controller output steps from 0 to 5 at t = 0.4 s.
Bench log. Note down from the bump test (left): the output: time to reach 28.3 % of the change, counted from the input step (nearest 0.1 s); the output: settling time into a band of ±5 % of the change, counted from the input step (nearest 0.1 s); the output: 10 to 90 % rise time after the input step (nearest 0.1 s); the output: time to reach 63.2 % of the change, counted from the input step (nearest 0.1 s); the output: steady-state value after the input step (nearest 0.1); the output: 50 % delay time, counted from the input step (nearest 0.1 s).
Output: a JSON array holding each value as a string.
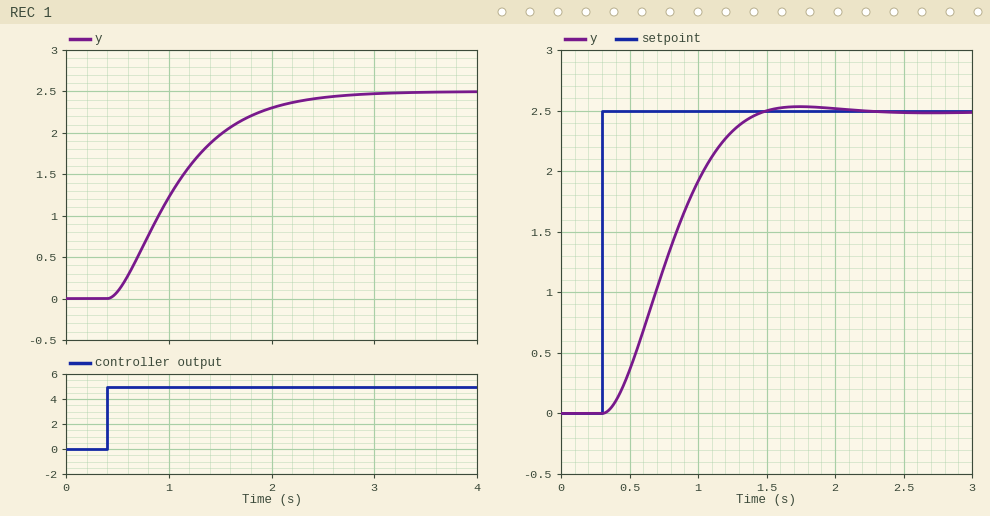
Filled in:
["0.4 s", "1.8 s", "1.3 s", "0.8 s", "2.5", "0.6 s"]
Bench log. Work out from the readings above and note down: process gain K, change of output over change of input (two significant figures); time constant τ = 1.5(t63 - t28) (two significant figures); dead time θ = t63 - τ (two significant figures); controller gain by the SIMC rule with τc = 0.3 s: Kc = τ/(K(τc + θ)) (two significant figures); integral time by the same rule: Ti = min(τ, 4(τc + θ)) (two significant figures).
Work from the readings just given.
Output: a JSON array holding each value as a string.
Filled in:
["0.50", "0.60 s", "0.20 s", "2.4", "0.60 s"]
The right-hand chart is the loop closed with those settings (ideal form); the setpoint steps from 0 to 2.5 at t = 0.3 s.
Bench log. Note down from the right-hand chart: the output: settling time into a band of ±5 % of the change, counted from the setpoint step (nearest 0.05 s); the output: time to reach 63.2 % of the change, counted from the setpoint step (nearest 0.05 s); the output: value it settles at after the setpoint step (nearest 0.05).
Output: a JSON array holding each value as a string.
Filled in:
["1.00 s", "0.55 s", "2.50"]
